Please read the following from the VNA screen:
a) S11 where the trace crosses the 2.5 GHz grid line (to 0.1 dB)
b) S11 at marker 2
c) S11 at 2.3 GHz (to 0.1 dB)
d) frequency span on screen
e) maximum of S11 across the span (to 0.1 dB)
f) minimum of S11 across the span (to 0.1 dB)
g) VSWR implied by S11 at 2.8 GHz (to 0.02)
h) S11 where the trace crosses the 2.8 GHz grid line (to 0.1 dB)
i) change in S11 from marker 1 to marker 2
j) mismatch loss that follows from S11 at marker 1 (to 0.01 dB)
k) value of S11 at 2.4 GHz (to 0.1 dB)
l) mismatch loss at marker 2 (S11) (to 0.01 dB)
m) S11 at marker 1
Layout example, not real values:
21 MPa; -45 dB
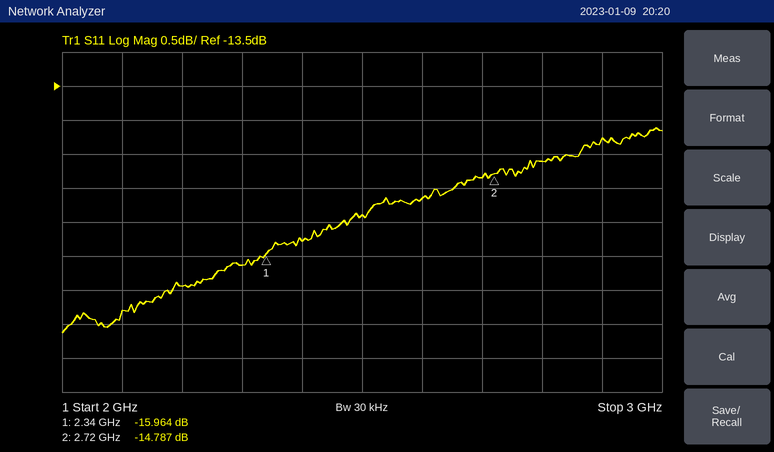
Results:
-15.4 dB; -14.787 dB; -16.1 dB; 1 GHz; -14.1 dB; -17.1 dB; 1.46; -14.6 dB; 1.177 dB; 0.11 dB; -15.8 dB; 0.15 dB; -15.964 dB
